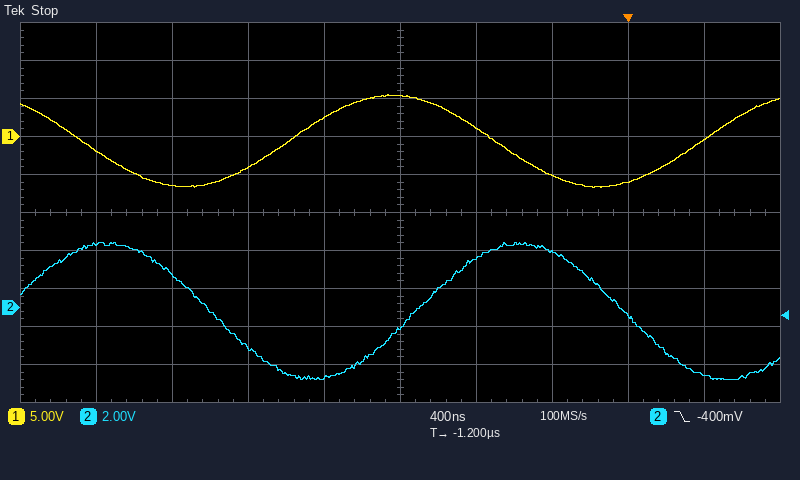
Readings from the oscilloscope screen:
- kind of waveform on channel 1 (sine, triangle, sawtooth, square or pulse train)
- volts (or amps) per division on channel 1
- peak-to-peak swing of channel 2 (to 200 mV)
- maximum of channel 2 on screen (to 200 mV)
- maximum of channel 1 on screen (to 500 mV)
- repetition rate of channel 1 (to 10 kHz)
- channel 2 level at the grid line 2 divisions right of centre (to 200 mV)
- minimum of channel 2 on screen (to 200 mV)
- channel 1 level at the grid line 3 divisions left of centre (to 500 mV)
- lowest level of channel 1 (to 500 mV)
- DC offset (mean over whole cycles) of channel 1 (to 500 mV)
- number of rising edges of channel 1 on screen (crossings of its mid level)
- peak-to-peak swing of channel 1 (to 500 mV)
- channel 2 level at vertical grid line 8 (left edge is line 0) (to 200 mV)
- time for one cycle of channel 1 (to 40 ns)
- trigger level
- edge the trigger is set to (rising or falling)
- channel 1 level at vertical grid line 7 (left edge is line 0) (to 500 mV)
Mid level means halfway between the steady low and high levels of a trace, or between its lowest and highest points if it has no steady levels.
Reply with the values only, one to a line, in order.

sine
5 V
7.2 V
3.4 V
5.5 V
460 kHz
3.0 V
-3.8 V
-6.5 V
-6.5 V
-500 mV
2
12.0 V
-400 mV
2.16 µs
-400 mV
falling
-5.0 V
